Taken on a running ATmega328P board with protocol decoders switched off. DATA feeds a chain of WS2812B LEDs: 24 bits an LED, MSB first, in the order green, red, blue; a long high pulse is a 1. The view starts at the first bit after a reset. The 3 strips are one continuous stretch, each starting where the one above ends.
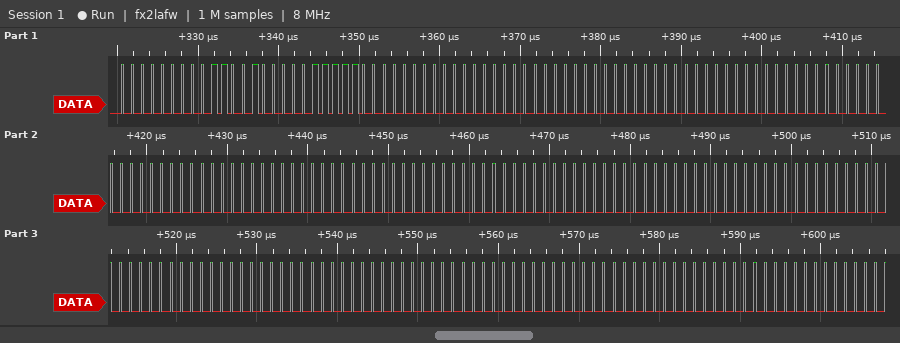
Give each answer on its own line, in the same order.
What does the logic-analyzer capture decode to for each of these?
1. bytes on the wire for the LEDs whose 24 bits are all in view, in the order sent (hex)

00 64 1F 00 00 00 00 00 00 00 00 00 00 00 00 00 00 00 00 00 00 00 00 00 00 00 00
